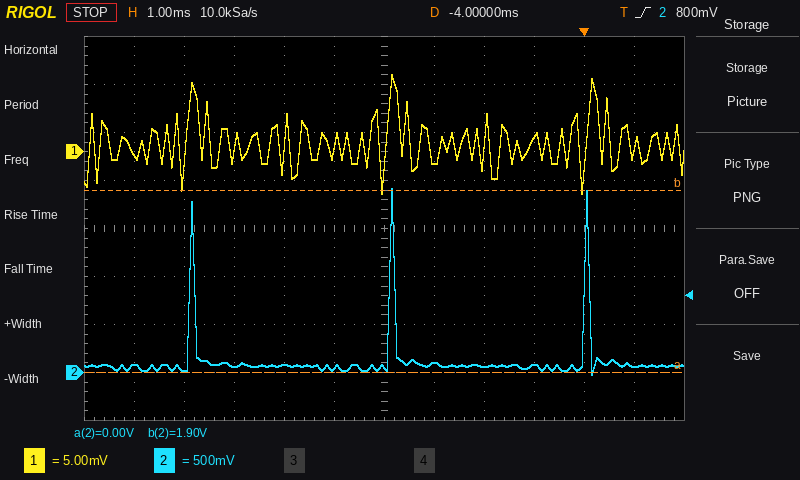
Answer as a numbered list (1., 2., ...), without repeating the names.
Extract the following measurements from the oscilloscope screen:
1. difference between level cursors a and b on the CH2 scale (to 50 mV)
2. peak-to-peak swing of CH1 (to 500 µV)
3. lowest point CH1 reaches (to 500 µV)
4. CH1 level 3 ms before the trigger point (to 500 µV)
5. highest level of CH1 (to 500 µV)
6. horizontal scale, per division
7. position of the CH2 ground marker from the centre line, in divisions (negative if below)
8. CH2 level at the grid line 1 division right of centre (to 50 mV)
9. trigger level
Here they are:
1. 1.90 V
2. 12.5 mV
3. -4.5 mV
4. -1.0 mV
5. 8.0 mV
6. 1 ms
7. -3.0 div
8. 100 mV
9. 800 mV
